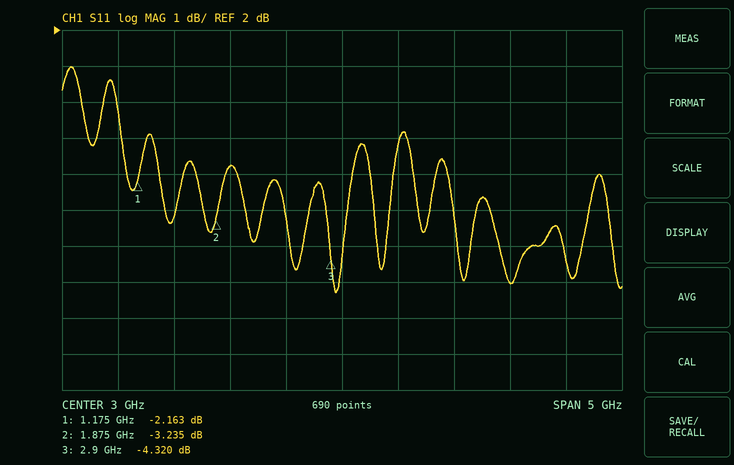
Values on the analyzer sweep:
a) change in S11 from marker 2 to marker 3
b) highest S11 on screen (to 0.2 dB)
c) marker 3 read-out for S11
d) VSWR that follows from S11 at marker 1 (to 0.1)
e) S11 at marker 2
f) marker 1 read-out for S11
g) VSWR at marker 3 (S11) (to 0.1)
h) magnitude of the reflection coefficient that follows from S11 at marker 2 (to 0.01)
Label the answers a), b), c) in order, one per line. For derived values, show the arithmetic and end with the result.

a) -4.32 − (-3.235) = -1.085 dB
b) 1.0 dB
c) -4.320 dB
d) (1 + 0.7796)/(1 − 0.7796) ≈ 8.1
e) -3.235 dB
f) -2.163 dB
g) (1 + 0.6081)/(1 − 0.6081) ≈ 4.1
h) 10^(-3.235/20) ≈ 0.69
